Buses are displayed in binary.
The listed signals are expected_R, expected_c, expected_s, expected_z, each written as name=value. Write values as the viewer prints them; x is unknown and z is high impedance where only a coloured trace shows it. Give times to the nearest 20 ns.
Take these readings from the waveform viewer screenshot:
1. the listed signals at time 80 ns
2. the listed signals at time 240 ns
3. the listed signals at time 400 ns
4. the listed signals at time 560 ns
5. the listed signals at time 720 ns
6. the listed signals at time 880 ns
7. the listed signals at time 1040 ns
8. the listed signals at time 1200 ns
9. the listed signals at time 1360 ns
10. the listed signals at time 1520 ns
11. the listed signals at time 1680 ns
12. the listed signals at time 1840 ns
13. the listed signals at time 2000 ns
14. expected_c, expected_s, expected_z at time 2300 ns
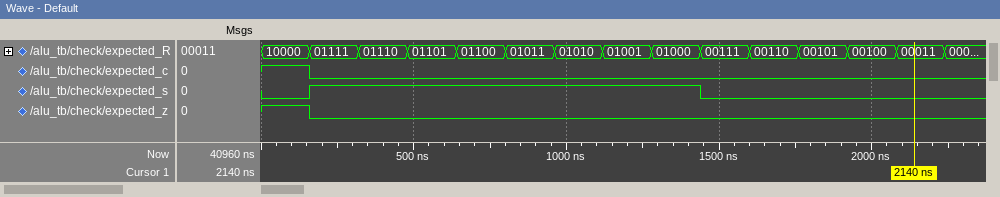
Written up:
expected_R=10000, expected_c=1, expected_s=0, expected_z=1
expected_R=01111, expected_c=0, expected_s=1, expected_z=0
expected_R=01110, expected_c=0, expected_s=1, expected_z=0
expected_R=01101, expected_c=0, expected_s=1, expected_z=0
expected_R=01100, expected_c=0, expected_s=1, expected_z=0
expected_R=01011, expected_c=0, expected_s=1, expected_z=0
expected_R=01010, expected_c=0, expected_s=1, expected_z=0
expected_R=01001, expected_c=0, expected_s=1, expected_z=0
expected_R=01000, expected_c=0, expected_s=1, expected_z=0
expected_R=00111, expected_c=0, expected_s=0, expected_z=0
expected_R=00110, expected_c=0, expected_s=0, expected_z=0
expected_R=00101, expected_c=0, expected_s=0, expected_z=0
expected_R=00100, expected_c=0, expected_s=0, expected_z=0
expected_c=0, expected_s=0, expected_z=0
